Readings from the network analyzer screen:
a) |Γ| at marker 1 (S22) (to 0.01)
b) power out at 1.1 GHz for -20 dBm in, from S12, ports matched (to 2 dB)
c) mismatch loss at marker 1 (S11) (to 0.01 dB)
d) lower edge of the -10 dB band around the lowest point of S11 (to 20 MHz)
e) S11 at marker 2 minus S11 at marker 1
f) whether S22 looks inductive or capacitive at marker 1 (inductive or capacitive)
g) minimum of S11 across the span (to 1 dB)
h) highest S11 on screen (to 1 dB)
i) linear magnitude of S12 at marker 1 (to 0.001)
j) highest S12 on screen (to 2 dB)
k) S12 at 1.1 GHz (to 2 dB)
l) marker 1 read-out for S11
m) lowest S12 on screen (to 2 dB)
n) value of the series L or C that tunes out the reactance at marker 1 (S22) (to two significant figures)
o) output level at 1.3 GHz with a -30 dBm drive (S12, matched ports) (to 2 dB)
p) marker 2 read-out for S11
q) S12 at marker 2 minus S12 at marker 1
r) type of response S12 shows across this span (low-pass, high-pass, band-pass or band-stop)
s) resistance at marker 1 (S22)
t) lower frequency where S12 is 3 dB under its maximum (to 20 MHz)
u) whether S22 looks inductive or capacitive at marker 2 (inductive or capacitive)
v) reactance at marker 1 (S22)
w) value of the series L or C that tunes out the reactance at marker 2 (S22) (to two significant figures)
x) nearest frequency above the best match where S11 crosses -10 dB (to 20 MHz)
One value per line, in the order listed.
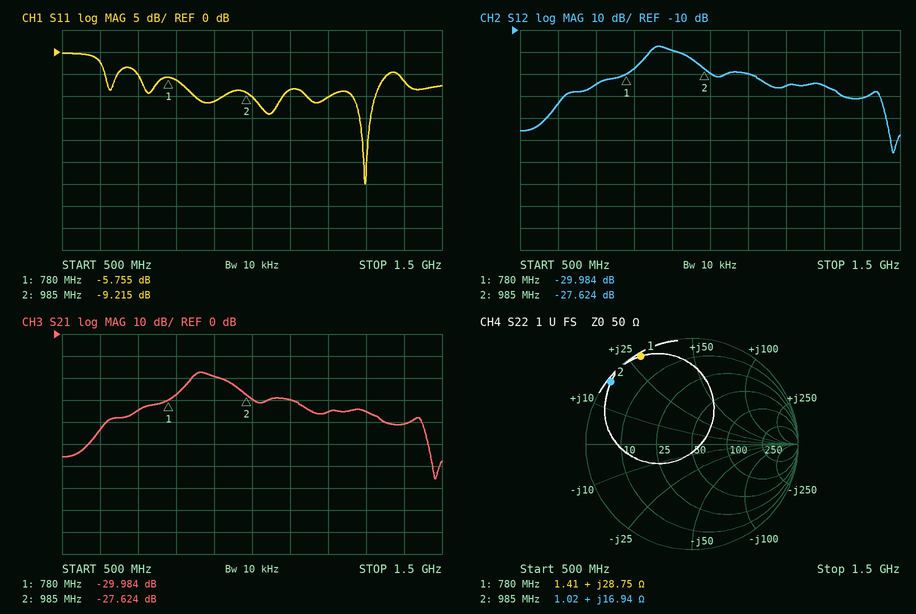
0.96
-50 dBm
1.34 dB
1.26 GHz
-3.460 dB
inductive
-30 dB
0 dB
0.032
-18 dB
-30 dB
-5.755 dB
-66 dB
7.1 pF
-66 dBm
-9.215 dB
2.360 dB
band-pass
1.41 Ω
840 MHz
inductive
+28.75 Ω
9.5 pF
1.32 GHz
